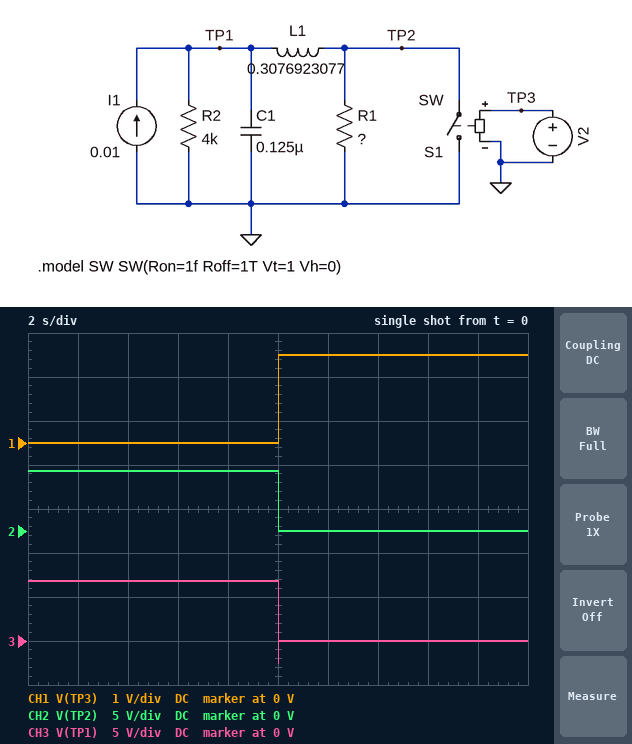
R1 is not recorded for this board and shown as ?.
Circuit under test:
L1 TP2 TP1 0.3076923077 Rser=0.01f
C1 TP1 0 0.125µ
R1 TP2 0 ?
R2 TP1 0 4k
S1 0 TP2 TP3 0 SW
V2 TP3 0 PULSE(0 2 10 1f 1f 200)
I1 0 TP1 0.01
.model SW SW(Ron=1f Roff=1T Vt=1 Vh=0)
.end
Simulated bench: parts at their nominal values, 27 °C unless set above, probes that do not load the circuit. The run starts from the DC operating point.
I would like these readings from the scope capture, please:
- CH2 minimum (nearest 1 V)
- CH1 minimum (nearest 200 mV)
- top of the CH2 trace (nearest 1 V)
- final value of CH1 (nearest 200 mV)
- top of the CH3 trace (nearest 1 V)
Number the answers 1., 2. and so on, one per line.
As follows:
1. 0 V
2. 0 V
3. 7 V
4. 2.0 V
5. 7 V
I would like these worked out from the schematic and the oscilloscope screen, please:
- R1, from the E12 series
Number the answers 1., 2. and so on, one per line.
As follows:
1. 820 Ω
